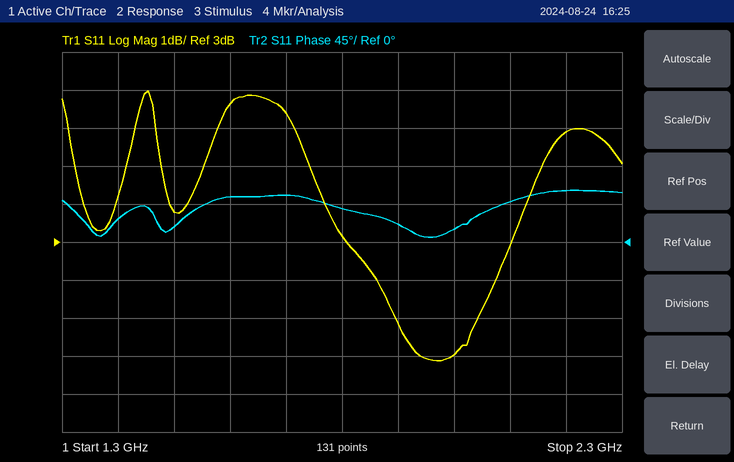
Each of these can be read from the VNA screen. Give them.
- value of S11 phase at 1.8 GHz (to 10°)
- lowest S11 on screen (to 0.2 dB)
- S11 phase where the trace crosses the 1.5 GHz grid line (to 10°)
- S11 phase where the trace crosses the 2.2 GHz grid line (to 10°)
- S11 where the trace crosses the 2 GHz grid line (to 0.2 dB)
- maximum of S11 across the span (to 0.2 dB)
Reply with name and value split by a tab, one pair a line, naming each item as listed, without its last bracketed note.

value of S11 phase at 1.8 GHz	40°
lowest S11 on screen	-0.2 dB
S11 phase where the trace crosses the 1.5 GHz grid line	20°
S11 phase where the trace crosses the 2.2 GHz grid line	60°
S11 where the trace crosses the 2 GHz grid line	0.0 dB
maximum of S11 across the span	7.0 dB
